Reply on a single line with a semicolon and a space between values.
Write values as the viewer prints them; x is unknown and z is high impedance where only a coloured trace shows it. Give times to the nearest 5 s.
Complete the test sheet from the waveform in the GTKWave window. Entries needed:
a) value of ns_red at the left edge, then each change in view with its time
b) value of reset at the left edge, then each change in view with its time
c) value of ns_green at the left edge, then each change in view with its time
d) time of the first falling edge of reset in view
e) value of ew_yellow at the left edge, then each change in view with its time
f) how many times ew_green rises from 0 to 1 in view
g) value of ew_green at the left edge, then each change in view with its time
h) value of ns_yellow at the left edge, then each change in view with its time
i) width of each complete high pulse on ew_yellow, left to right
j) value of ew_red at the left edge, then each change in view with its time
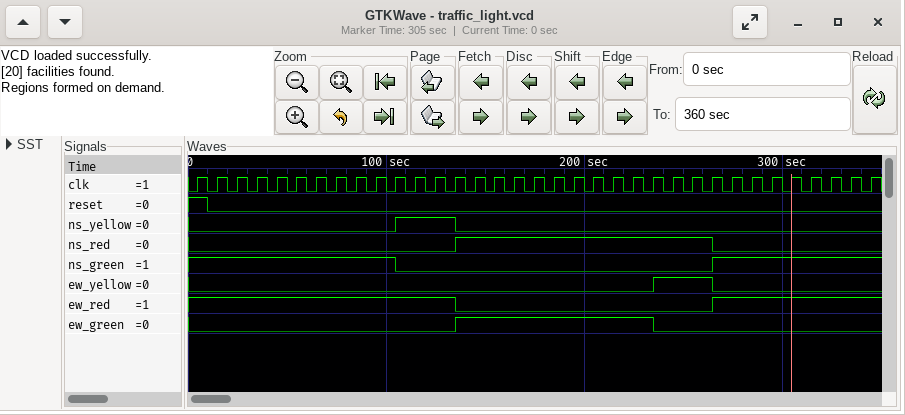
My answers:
0, 1 at 135 s, 0 at 265 s; 1, 0 at 10 s; 1, 0 at 105 s, 1 at 265 s; 10 s; 0, 1 at 235 s, 0 at 265 s; 1; 0, 1 at 135 s, 0 at 235 s; 0, 1 at 105 s, 0 at 135 s; 30 s; 1, 0 at 135 s, 1 at 265 s
